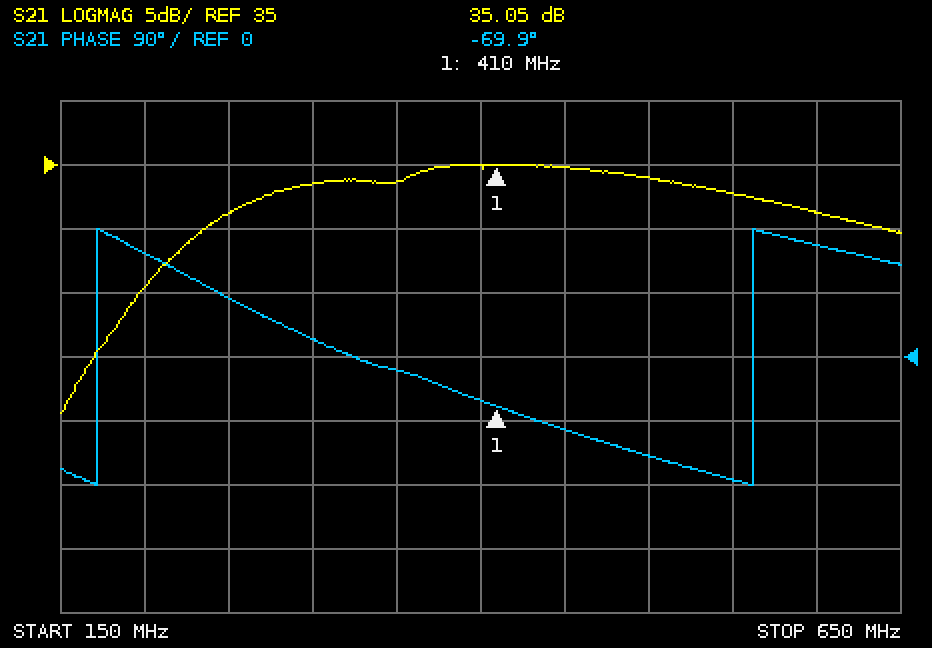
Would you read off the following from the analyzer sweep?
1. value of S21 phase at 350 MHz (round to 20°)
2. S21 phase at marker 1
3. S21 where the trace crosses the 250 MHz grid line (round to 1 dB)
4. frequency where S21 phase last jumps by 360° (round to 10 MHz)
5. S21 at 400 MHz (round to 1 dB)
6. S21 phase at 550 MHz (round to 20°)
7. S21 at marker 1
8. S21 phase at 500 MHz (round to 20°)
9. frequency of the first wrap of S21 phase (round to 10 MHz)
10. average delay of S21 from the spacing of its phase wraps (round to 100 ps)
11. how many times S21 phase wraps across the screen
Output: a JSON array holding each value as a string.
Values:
["-20°", "-69.9°", "31 dB", "560 MHz", "35 dB", "-180°", "35.05 dB", "-140°", "170 MHz", "2.6 ns", "2"]
